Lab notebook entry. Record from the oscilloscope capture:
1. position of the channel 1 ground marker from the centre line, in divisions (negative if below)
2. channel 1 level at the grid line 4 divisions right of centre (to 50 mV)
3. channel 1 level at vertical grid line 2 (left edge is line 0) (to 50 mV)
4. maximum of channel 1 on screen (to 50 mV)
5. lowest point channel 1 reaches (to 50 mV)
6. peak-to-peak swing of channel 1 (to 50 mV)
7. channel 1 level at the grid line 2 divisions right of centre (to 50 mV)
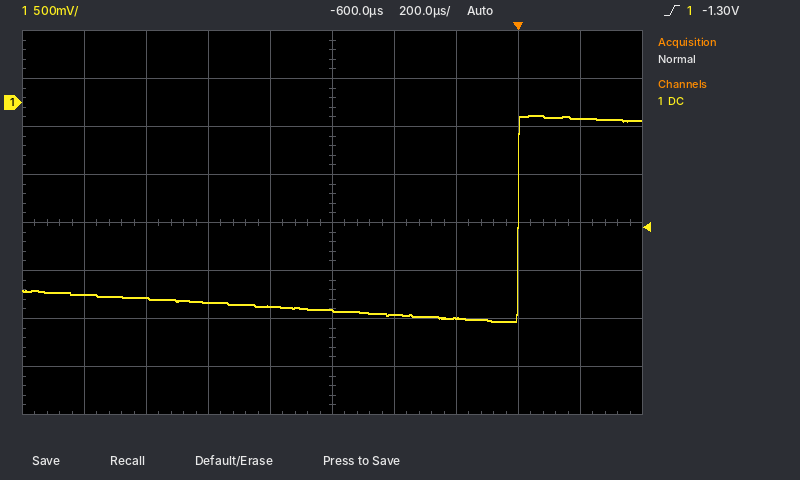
+2.5 div
-150 mV
-2.05 V
-150 mV
-2.30 V
2.15 V
-2.25 V
